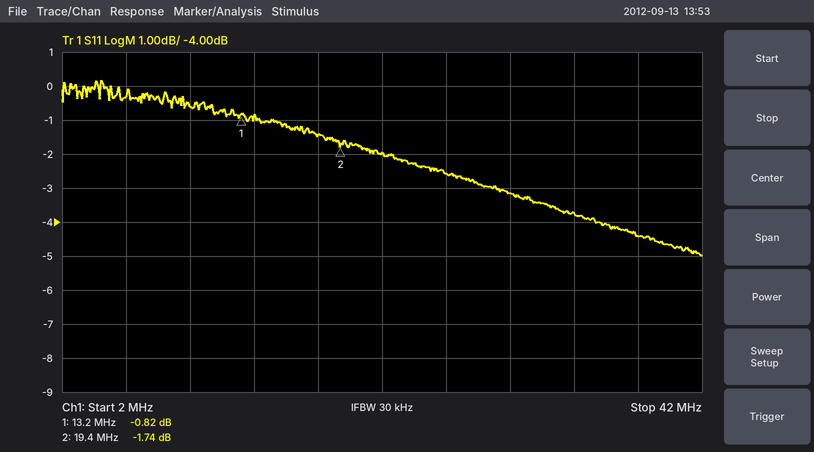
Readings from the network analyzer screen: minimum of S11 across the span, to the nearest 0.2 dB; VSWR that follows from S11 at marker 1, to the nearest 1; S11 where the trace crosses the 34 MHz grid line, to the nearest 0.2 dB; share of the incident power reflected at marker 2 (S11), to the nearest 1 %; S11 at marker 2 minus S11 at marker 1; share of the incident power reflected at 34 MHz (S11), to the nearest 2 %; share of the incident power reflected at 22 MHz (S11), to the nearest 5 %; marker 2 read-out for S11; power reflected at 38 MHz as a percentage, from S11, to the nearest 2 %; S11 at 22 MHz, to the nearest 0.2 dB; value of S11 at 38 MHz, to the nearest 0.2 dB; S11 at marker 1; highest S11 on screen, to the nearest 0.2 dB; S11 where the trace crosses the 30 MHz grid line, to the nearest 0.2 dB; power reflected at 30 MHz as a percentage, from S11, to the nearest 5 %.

-5.0 dB
21
-3.8 dB
67 %
-0.92 dB
42 %
65 %
-1.74 dB
36 %
-2.0 dB
-4.4 dB
-0.82 dB
0.2 dB
-3.2 dB
50 %
